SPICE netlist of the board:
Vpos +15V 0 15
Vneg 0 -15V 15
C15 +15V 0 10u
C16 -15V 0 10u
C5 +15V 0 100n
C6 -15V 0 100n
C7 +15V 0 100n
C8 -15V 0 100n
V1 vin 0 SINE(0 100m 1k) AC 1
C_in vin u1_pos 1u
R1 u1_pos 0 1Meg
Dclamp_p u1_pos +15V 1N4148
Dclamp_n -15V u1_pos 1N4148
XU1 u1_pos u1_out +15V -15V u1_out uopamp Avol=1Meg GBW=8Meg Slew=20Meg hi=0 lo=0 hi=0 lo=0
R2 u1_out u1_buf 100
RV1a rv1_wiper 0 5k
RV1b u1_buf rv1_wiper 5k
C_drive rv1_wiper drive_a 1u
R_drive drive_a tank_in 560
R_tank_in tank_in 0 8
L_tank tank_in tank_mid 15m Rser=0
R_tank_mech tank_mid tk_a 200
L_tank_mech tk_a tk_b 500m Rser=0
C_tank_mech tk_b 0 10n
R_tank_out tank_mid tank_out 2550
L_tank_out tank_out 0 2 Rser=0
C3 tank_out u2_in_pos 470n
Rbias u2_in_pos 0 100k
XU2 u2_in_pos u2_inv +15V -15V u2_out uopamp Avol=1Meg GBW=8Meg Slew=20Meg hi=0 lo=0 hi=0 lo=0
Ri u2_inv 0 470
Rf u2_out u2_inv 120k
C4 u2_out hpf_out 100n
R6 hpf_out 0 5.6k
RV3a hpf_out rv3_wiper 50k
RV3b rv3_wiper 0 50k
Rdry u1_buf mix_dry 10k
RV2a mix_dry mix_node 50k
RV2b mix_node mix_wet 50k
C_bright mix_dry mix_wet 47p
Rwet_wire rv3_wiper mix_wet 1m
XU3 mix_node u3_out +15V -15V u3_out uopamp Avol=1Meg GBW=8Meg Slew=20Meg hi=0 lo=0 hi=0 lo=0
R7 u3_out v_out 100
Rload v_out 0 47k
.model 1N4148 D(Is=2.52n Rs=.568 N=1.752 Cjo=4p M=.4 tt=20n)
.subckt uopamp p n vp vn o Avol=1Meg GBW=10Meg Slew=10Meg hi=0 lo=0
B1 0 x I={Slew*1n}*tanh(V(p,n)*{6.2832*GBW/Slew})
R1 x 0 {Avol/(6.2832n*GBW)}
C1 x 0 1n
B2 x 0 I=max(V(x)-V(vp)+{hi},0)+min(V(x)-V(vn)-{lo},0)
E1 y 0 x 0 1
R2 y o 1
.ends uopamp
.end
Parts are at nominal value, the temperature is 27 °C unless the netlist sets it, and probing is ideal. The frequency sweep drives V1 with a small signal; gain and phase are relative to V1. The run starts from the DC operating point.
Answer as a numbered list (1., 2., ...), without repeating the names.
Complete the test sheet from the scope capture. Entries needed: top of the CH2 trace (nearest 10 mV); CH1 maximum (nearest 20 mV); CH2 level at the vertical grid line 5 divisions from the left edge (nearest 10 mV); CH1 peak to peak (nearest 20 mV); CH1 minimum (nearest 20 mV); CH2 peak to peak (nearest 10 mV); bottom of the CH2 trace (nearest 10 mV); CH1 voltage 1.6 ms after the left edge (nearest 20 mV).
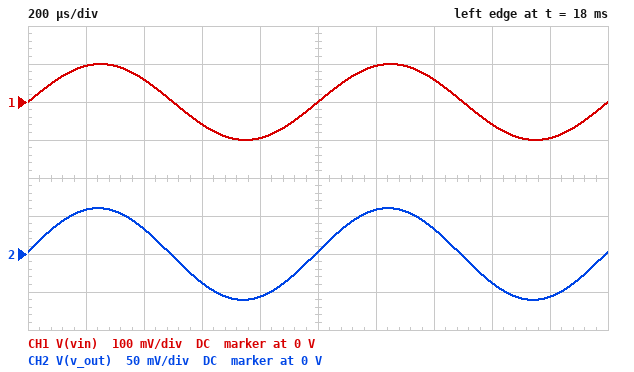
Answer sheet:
1. 60 mV
2. 100 mV
3. 0 V
4. 200 mV
5. -100 mV
6. 120 mV
7. -60 mV
8. -60 mV
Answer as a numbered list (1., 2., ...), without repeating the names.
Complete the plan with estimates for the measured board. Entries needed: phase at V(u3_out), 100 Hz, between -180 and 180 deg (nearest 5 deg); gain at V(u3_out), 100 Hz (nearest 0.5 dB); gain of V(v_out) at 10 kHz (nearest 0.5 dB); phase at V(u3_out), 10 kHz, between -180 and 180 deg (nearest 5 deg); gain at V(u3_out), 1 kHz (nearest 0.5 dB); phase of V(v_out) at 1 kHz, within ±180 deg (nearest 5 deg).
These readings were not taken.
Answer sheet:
1. 0 deg
2. -5.5 dB
3. -4.5 dB
4. 0 deg
5. -4.5 dB
6. 5 deg
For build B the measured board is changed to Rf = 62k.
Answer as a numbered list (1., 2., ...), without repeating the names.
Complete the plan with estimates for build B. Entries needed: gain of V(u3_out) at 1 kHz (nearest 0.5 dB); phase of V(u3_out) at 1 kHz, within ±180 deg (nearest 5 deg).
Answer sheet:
1. -5.0 dB
2. 0 deg
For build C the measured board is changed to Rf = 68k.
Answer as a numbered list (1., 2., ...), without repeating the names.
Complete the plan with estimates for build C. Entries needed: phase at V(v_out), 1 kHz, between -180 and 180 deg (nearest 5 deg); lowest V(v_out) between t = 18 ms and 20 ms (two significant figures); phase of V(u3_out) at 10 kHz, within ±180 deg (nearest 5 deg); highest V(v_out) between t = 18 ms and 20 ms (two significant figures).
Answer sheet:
1. 0 deg
2. -58 mV
3. 0 deg
4. 58 mV
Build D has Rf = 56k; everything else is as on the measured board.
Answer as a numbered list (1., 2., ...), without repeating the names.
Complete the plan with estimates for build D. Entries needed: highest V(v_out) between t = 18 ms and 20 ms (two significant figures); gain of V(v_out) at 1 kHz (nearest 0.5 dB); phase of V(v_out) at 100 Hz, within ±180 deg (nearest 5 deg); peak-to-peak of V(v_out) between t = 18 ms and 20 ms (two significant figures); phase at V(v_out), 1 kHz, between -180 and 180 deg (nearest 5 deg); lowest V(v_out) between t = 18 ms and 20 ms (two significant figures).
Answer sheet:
1. 57 mV
2. -5.0 dB
3. 0 deg
4. 110 mV
5. 0 deg
6. -57 mV
